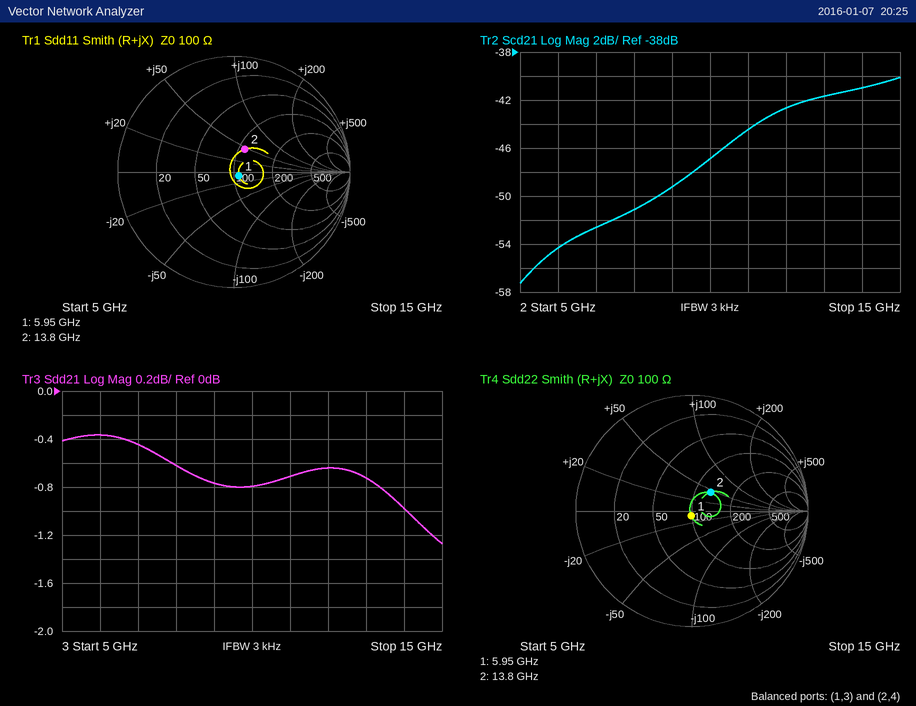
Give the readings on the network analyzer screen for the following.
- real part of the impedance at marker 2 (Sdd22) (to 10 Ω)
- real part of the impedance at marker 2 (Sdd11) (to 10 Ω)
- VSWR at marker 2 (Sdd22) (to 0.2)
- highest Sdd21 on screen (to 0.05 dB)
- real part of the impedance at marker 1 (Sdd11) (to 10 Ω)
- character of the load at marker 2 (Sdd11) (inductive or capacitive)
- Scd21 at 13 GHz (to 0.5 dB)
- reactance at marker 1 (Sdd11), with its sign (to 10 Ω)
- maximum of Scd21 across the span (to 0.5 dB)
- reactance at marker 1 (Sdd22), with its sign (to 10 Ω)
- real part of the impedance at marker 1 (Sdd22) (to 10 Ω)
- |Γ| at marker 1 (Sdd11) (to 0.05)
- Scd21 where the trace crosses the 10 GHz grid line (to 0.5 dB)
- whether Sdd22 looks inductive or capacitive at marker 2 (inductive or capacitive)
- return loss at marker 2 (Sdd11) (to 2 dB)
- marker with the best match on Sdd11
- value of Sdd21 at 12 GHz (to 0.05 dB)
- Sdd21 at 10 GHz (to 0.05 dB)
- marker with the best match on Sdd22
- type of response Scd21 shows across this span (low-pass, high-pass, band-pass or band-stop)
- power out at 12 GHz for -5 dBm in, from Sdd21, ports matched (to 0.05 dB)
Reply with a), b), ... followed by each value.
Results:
a) 130 Ω
b) 110 Ω
c) 1.6
d) -0.35 dB
e) 110 Ω
f) inductive
g) -41.5 dB
h) -10 Ω
i) -40.0 dB
j) -10 Ω
k) 100 Ω
l) 0.05
m) -47.0 dB
n) inductive
o) 14 dB
p) marker 1
q) -0.65 dB
r) -0.80 dB
s) marker 1
t) high-pass
u) -5.65 dBm
